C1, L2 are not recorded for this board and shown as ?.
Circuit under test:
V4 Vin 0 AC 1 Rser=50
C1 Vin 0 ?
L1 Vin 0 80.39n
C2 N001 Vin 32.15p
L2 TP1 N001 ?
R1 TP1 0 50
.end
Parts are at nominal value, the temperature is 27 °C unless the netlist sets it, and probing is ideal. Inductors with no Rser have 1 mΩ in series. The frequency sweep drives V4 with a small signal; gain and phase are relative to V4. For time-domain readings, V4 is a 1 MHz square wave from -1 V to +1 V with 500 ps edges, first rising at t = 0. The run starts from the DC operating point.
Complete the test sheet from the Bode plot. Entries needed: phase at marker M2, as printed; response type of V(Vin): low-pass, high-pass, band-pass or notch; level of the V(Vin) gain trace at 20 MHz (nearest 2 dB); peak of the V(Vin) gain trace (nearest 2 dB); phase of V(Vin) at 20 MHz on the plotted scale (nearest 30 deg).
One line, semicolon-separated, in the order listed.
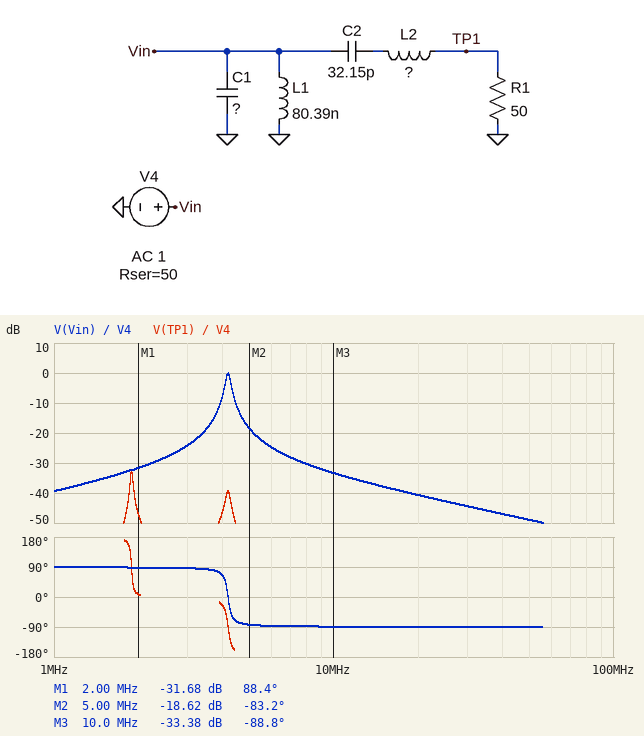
-83.2 deg; band-pass; -40 dB; 0 dB; -90 deg
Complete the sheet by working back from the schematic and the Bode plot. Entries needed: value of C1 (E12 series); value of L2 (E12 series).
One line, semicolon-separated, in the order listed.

18 nF; 220 µH
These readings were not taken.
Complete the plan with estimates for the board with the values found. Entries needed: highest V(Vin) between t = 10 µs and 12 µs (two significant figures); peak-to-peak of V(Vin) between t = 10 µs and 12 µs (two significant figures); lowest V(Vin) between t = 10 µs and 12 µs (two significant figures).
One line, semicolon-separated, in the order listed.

48 mV; 97 mV; -48 mV
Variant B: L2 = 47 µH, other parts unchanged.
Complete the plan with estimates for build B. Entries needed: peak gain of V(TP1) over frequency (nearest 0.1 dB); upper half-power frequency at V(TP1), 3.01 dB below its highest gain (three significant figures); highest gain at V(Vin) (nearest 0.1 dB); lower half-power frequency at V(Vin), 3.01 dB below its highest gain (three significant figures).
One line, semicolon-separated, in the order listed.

-7.1 dB; 4.28 MHz; -2.2 dB; 4.16 MHz
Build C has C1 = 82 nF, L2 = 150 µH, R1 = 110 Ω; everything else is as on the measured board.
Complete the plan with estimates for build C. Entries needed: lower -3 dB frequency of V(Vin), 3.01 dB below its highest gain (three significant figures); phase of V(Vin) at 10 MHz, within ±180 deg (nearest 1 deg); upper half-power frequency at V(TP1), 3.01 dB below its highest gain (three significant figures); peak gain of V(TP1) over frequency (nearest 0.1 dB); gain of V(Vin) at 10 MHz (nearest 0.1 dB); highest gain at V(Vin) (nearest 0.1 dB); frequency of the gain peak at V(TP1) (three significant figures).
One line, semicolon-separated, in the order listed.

1.94 MHz; -90 deg; 1.98 MHz; -16.5 dB; -47.9 dB; -0.5 dB; 1.96 MHz
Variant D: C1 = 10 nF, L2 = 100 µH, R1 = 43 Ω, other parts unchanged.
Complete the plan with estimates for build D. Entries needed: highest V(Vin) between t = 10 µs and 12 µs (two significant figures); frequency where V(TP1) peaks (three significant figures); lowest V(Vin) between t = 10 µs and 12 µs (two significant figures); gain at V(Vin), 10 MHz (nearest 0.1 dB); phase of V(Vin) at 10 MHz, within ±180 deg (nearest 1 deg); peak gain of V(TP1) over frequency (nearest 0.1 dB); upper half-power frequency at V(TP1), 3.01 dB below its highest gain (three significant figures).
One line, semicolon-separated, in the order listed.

82 mV; 2.81 MHz; -82 mV; -26.7 dB; -87 deg; -28.5 dB; 2.84 MHz
